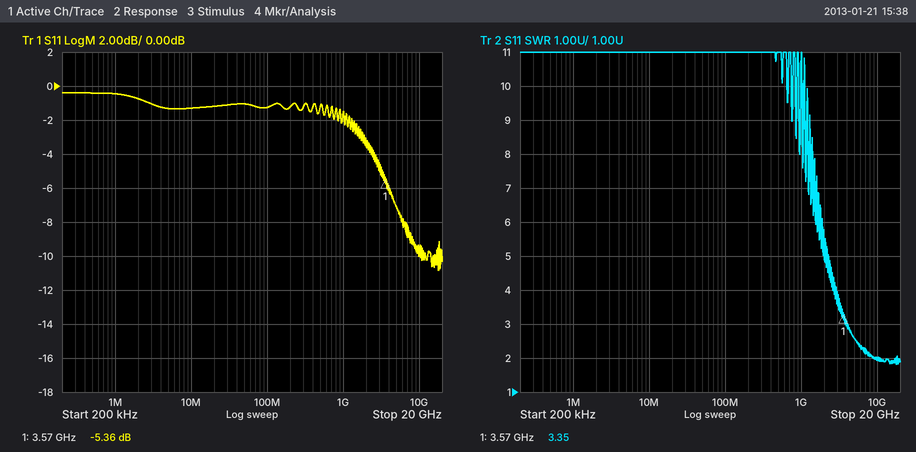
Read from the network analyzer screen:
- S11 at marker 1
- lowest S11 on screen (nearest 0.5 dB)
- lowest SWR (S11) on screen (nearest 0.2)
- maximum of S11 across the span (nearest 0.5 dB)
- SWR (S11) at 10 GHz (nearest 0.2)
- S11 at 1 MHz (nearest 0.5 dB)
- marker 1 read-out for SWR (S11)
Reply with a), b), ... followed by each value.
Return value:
a) -5.36 dB
b) -11.0 dB
c) 1.8
d) -0.5 dB
e) 2.0
f) -0.5 dB
g) 3.35
